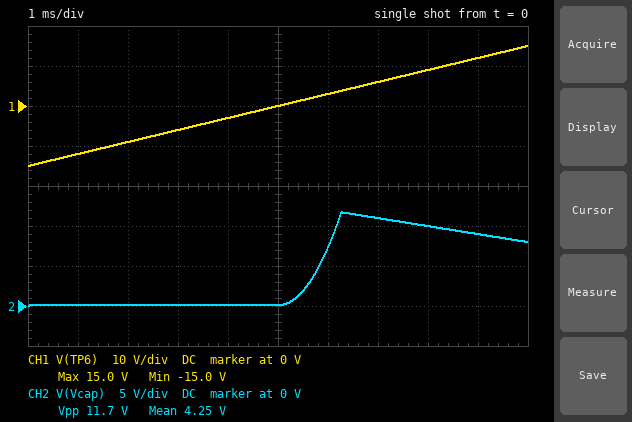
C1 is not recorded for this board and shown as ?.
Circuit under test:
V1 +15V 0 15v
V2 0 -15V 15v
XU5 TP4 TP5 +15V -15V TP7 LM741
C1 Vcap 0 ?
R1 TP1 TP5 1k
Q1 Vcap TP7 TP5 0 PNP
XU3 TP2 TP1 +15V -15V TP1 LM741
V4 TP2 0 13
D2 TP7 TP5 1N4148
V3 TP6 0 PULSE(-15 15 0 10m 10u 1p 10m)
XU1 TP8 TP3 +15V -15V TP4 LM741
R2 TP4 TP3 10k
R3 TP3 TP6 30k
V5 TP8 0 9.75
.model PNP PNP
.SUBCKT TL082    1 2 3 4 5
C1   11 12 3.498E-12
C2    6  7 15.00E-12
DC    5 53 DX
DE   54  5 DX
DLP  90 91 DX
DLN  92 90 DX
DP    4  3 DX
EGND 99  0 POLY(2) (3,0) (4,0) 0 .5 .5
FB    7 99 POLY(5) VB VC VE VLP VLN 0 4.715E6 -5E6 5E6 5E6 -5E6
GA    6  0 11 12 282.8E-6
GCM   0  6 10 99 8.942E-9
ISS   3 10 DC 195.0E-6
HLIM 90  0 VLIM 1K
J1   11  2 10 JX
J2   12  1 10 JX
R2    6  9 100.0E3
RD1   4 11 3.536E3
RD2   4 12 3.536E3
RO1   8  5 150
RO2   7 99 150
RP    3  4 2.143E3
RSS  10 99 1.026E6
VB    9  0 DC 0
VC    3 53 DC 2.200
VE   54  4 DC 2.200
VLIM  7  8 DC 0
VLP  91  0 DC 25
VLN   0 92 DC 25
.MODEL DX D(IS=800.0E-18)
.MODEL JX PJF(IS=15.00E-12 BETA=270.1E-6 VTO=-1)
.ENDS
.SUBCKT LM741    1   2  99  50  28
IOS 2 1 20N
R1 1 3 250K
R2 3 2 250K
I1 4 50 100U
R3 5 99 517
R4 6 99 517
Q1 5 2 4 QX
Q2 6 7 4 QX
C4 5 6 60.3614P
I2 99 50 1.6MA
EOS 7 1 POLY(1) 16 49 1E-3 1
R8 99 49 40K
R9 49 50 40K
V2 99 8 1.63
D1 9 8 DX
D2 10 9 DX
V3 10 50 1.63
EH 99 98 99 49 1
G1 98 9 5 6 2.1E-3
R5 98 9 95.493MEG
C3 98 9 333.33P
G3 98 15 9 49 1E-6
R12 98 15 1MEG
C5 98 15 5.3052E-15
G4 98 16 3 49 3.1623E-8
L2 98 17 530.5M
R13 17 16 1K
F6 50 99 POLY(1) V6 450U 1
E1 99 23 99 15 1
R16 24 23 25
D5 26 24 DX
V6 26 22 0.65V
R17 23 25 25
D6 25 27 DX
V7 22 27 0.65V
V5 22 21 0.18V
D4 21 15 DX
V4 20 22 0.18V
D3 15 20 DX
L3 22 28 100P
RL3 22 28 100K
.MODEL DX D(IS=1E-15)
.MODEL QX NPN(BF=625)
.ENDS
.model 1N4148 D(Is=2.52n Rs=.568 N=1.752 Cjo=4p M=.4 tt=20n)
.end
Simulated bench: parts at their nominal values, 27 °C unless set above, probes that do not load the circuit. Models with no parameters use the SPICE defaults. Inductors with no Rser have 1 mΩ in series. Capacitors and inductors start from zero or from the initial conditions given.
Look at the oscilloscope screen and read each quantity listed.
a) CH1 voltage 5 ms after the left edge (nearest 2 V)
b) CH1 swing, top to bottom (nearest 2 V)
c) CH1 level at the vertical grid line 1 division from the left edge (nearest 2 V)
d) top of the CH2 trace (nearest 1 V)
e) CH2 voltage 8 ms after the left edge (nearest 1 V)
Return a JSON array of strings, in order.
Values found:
["0 V", "30 V", "-12 V", "12 V", "10 V"]
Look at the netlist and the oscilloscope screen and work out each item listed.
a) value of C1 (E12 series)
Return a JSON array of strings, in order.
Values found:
["68 nF"]
